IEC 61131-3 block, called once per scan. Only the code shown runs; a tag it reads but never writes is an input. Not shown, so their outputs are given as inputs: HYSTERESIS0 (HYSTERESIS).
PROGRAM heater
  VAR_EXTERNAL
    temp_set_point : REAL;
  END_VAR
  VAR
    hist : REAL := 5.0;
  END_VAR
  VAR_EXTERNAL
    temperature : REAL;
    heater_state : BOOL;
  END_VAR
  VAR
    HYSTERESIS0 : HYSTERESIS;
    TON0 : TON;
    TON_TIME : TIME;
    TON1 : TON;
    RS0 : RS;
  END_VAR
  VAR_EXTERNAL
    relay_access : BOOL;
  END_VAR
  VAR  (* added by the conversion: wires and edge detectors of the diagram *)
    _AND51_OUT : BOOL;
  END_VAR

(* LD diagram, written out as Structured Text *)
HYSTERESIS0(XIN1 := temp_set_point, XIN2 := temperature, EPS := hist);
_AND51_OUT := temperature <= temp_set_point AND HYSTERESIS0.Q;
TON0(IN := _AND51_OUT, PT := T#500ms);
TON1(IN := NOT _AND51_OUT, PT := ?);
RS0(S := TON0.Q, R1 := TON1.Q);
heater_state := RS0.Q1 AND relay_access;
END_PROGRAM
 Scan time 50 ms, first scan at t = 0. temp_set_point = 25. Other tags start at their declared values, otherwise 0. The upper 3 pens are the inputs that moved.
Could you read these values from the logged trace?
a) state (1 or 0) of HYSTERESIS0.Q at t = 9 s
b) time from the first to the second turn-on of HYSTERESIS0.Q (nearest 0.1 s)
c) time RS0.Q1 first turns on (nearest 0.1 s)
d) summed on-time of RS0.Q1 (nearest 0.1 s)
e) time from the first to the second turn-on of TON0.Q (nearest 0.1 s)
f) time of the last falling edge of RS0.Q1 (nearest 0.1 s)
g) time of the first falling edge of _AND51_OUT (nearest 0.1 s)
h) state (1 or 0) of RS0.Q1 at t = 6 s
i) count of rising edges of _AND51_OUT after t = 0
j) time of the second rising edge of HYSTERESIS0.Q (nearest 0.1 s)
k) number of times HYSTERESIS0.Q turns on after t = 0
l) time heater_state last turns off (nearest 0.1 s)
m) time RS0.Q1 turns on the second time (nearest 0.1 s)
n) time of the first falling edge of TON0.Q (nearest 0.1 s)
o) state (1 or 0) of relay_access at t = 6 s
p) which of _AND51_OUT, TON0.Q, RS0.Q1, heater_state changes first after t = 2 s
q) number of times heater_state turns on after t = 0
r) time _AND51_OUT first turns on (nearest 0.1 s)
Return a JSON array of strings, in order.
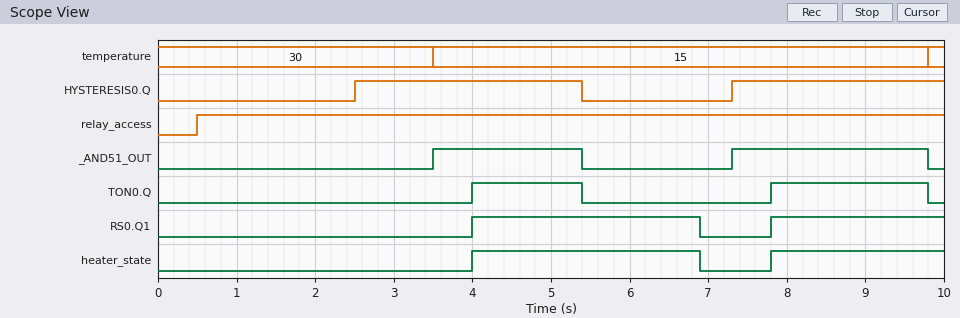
["1", "4.8 s", "4.0 s", "5.1 s", "3.8 s", "6.9 s", "5.4 s", "1", "2", "7.3 s", "2", "6.9 s", "7.8 s", "5.4 s", "1", "_AND51_OUT", "2", "3.5 s"]
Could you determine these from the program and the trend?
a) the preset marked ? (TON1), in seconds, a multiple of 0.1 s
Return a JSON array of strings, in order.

["1.5 s"]
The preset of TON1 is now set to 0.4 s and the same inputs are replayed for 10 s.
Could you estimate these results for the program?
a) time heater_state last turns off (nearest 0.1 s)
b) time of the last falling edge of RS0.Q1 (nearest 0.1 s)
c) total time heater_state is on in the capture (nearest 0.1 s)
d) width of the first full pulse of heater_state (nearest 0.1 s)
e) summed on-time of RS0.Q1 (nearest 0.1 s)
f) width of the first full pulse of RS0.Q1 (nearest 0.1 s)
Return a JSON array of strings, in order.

["5.8 s", "5.8 s", "4.0 s", "1.8 s", "4.0 s", "1.8 s"]
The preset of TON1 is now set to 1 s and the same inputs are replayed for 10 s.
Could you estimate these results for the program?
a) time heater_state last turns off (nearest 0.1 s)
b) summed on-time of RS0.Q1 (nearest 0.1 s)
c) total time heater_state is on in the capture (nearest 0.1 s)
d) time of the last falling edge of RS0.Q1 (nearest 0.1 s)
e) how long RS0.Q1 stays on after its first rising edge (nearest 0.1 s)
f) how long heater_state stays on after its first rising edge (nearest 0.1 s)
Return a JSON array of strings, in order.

["6.4 s", "4.6 s", "4.6 s", "6.4 s", "2.4 s", "2.4 s"]
